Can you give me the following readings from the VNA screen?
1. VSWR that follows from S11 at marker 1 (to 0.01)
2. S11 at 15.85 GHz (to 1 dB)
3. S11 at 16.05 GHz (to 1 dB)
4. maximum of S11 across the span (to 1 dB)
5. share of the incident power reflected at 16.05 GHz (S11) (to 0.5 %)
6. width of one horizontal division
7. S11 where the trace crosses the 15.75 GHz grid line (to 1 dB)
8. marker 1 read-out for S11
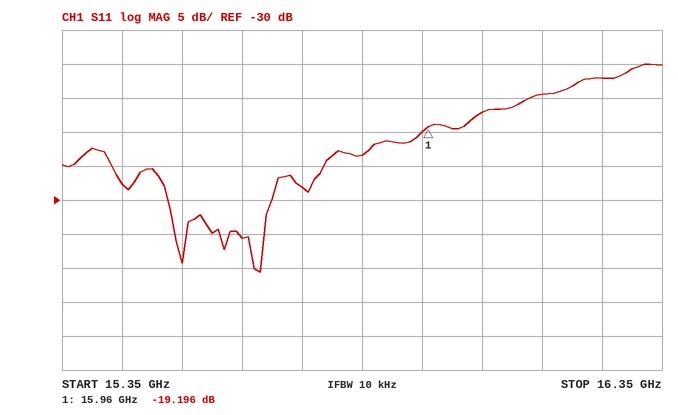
1.25
-23 dB
-17 dB
-10 dB
2.0 %
100 MHz
-28 dB
-19.196 dB
